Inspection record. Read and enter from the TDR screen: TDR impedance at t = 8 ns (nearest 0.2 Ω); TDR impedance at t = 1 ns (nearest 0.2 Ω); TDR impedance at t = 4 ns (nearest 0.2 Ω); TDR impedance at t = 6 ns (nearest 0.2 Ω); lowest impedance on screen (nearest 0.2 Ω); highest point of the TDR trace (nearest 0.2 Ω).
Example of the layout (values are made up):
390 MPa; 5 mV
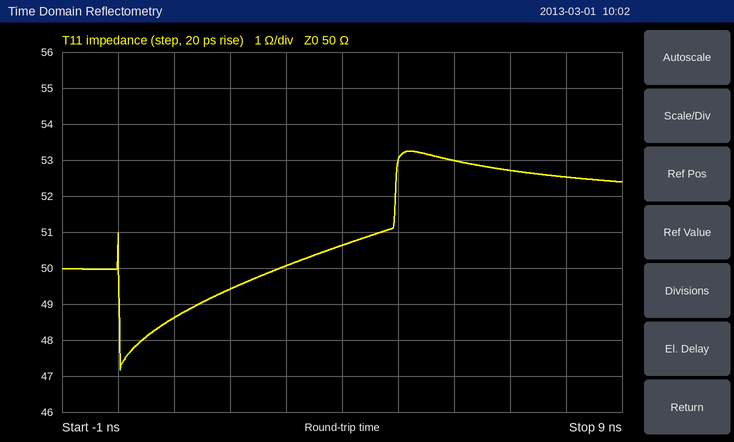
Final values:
52.6 Ω; 48.6 Ω; 50.6 Ω; 53.0 Ω; 47.2 Ω; 53.2 Ω
